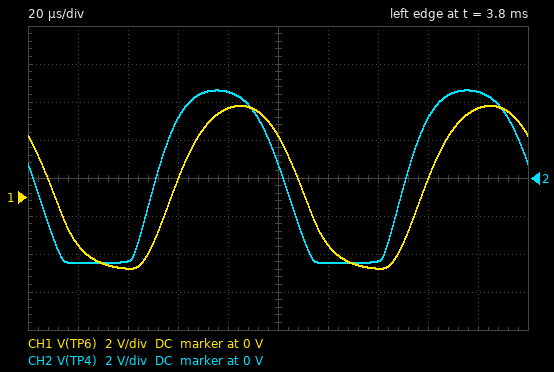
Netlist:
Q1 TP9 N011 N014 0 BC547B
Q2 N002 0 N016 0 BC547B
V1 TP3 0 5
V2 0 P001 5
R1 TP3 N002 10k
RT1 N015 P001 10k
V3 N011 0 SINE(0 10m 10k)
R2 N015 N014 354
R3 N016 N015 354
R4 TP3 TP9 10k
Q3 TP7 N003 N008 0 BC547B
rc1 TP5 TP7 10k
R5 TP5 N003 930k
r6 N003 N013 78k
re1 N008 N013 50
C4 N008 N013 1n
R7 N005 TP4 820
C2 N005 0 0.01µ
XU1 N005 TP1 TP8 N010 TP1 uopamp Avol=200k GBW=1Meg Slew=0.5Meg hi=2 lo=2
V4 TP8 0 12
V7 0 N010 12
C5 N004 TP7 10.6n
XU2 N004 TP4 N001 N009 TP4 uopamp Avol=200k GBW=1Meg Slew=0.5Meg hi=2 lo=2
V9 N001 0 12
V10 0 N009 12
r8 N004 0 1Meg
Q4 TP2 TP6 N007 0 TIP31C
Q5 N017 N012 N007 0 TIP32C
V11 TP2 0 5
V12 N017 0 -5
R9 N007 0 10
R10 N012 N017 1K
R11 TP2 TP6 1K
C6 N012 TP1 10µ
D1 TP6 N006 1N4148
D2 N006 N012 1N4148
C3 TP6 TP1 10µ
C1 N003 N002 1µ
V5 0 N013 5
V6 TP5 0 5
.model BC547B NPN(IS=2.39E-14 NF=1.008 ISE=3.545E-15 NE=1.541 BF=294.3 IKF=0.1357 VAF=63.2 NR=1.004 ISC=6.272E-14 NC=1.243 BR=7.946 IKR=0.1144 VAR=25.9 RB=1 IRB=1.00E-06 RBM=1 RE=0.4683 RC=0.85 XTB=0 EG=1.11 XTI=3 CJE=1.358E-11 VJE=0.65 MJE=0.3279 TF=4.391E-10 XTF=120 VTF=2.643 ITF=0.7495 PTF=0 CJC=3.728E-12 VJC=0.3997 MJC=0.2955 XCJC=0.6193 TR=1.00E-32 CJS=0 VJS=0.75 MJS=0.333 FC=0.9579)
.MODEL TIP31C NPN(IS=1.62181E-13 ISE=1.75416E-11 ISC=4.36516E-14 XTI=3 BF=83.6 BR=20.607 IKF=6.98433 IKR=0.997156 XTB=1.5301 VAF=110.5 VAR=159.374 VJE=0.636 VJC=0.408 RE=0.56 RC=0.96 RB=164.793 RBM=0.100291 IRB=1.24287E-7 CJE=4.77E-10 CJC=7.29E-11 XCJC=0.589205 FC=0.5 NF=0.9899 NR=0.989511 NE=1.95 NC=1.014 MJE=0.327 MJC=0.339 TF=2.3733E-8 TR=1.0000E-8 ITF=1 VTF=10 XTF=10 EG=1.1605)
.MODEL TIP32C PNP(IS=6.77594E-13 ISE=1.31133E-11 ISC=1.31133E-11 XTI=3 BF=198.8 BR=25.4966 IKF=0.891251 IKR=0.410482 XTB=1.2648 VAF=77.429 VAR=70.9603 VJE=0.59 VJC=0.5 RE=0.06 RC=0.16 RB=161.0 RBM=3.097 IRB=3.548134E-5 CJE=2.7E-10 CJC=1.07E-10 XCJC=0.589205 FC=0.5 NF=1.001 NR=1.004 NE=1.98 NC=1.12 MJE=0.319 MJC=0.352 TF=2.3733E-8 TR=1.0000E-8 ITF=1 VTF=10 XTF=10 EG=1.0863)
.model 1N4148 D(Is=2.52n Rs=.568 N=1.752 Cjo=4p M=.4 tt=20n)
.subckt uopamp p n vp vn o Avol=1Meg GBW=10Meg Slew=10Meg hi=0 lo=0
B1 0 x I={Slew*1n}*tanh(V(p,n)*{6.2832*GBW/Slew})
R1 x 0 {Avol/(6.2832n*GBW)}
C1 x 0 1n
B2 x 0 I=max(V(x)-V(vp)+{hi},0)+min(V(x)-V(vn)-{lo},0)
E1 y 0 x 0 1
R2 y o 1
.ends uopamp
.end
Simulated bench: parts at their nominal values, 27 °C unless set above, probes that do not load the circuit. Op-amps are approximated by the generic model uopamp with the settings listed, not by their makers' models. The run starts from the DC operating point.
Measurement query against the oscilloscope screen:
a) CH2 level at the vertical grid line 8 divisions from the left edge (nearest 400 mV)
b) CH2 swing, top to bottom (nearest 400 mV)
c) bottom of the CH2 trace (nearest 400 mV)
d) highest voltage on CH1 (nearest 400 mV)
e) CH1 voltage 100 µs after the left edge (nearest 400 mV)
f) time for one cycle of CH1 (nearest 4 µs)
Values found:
3.2 V
9.2 V
-4.4 V
4.8 V
3.2 V
100 µs
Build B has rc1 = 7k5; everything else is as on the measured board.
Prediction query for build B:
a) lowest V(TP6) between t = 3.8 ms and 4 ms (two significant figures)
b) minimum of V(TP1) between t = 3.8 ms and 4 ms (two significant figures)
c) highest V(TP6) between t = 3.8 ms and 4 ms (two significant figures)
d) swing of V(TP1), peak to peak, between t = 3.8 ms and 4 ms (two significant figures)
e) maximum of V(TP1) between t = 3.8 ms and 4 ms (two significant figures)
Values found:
-4.1 V
-4.8 V
4.1 V
8.1 V
3.3 V
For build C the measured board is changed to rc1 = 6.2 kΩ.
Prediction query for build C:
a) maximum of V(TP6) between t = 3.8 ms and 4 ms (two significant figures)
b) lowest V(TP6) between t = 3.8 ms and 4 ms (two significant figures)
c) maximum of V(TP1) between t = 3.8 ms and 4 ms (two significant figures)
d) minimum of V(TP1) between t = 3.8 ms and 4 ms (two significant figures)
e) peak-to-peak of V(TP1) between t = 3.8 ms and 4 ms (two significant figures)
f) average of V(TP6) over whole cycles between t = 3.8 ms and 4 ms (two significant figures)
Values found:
3.5 V
-3.3 V
2.8 V
-4.0 V
6.8 V
410 mV
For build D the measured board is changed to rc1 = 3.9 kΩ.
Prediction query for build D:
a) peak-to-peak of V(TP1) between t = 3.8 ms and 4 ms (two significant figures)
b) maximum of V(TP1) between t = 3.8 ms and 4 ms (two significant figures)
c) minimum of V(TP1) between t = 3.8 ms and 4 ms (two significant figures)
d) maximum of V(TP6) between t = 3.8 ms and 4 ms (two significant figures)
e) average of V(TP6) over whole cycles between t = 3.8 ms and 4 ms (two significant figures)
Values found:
4.4 V
1.8 V
-2.6 V
2.5 V
470 mV
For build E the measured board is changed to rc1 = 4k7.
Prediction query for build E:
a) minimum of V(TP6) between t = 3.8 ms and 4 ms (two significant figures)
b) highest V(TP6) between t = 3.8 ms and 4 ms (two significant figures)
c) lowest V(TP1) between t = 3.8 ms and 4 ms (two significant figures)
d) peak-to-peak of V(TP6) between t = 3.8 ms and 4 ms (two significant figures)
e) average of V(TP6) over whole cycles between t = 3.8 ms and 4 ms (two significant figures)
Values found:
-2.4 V
2.8 V
-3.1 V
5.3 V
450 mV
